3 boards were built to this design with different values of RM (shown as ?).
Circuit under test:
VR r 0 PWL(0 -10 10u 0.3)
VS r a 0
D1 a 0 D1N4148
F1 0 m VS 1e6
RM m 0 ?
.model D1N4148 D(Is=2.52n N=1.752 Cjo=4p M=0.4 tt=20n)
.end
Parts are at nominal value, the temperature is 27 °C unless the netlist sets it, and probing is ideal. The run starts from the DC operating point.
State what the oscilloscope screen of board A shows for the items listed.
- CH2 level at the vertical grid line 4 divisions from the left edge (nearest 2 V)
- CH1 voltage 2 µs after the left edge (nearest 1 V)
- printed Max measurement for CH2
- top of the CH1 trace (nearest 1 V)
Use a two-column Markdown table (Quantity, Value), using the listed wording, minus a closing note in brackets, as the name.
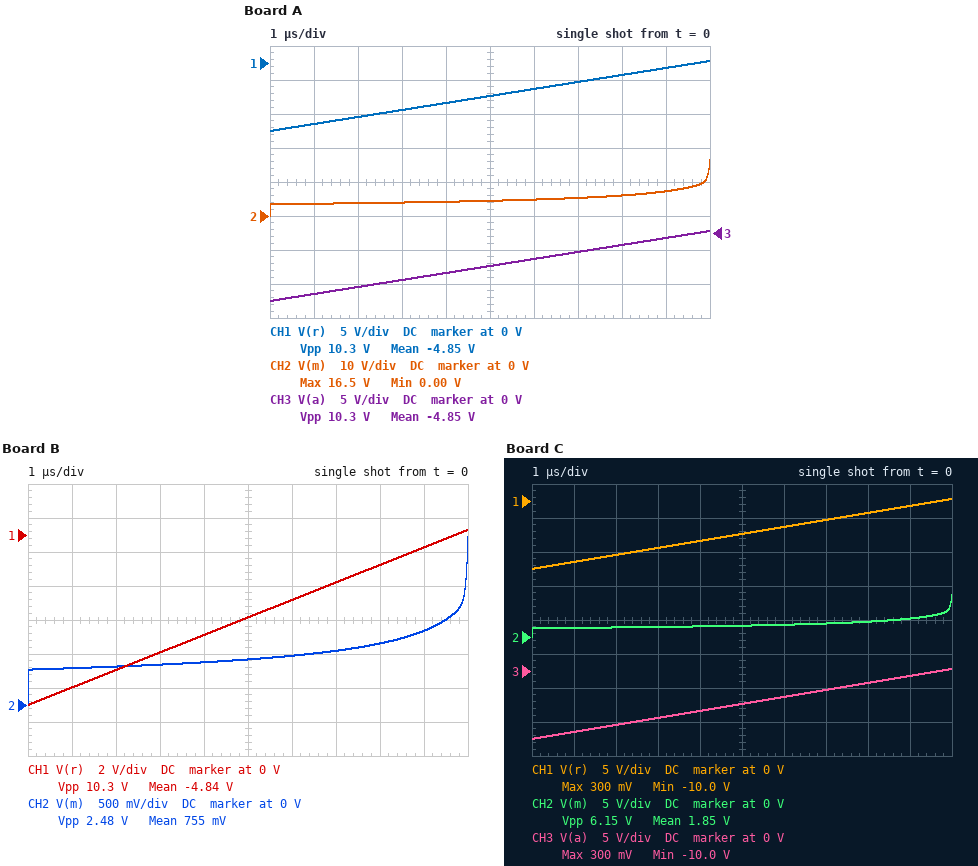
| Quantity | Value |
|---|---|
| CH2 level at the vertical grid line 4 divisions from the left edge | 4 V |
| CH1 voltage 2 µs after the left edge | -8 V |
| printed Max measurement for CH2 | 16.5 V |
| top of the CH1 trace | 0 V |
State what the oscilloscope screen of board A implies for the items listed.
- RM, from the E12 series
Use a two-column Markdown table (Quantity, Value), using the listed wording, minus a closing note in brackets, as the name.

| Quantity | Value |
|---|---|
| RM, from the E12 series | 2.2 Ω |
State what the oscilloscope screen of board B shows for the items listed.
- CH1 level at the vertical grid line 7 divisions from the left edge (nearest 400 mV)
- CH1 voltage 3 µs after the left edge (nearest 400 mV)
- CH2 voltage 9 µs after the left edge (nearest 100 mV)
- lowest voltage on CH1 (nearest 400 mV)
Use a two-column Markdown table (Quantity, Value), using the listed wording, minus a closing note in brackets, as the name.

| Quantity | Value |
|---|---|
| CH1 level at the vertical grid line 7 divisions from the left edge | -2.8 V |
| CH1 voltage 3 µs after the left edge | -6.8 V |
| CH2 voltage 9 µs after the left edge | 1.1 V |
| lowest voltage on CH1 | -10.0 V |
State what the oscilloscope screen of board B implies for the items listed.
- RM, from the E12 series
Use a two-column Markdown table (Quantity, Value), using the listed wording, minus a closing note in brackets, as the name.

| Quantity | Value |
|---|---|
| RM, from the E12 series | 0.33 Ω |
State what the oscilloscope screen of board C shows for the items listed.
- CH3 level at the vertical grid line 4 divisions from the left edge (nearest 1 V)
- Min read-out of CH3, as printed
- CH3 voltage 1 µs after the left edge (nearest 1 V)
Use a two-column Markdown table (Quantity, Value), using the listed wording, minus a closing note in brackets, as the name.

| Quantity | Value |
|---|---|
| CH3 level at the vertical grid line 4 divisions from the left edge | -6 V |
| Min read-out of CH3, as printed | -10.0 V |
| CH3 voltage 1 µs after the left edge | -9 V |
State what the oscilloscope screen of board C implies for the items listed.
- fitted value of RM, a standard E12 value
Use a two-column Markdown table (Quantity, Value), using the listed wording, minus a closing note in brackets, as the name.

| Quantity | Value |
|---|---|
| fitted value of RM, a standard E12 value | 0.82 Ω |
